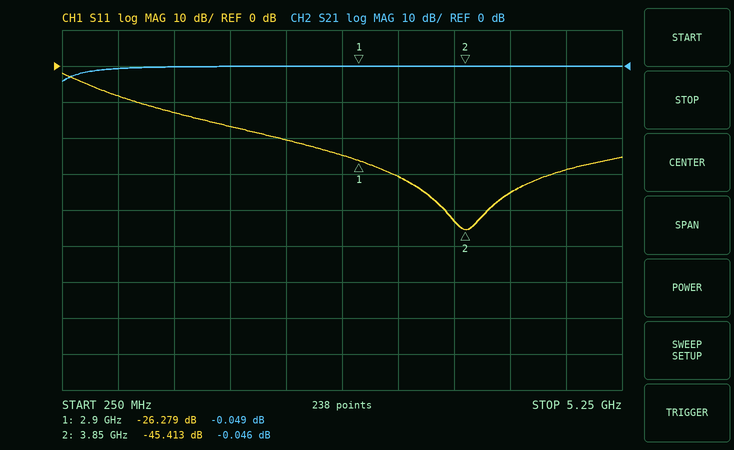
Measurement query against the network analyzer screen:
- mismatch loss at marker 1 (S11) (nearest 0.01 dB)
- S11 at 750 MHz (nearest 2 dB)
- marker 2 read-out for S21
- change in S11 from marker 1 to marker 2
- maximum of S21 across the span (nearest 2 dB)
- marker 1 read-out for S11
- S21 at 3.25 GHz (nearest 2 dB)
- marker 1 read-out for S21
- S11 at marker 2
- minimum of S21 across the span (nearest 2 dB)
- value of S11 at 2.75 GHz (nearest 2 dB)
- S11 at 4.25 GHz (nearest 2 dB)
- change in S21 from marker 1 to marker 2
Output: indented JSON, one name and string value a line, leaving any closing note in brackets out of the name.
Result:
{
  "mismatch loss at marker 1 (S11)": "0.01 dB",
  "S11 at 750 MHz": "-8 dB",
  "marker 2 read-out for S21": "-0.046 dB",
  "change in S11 from marker 1 to marker 2": "-19.134 dB",
  "maximum of S21 across the span": "0 dB",
  "marker 1 read-out for S11": "-26.279 dB",
  "S21 at 3.25 GHz": "0 dB",
  "marker 1 read-out for S21": "-0.049 dB",
  "S11 at marker 2": "-45.413 dB",
  "minimum of S21 across the span": "-4 dB",
  "value of S11 at 2.75 GHz": "-24 dB",
  "S11 at 4.25 GHz": "-36 dB",
  "change in S21 from marker 1 to marker 2": "0.003 dB"
}
